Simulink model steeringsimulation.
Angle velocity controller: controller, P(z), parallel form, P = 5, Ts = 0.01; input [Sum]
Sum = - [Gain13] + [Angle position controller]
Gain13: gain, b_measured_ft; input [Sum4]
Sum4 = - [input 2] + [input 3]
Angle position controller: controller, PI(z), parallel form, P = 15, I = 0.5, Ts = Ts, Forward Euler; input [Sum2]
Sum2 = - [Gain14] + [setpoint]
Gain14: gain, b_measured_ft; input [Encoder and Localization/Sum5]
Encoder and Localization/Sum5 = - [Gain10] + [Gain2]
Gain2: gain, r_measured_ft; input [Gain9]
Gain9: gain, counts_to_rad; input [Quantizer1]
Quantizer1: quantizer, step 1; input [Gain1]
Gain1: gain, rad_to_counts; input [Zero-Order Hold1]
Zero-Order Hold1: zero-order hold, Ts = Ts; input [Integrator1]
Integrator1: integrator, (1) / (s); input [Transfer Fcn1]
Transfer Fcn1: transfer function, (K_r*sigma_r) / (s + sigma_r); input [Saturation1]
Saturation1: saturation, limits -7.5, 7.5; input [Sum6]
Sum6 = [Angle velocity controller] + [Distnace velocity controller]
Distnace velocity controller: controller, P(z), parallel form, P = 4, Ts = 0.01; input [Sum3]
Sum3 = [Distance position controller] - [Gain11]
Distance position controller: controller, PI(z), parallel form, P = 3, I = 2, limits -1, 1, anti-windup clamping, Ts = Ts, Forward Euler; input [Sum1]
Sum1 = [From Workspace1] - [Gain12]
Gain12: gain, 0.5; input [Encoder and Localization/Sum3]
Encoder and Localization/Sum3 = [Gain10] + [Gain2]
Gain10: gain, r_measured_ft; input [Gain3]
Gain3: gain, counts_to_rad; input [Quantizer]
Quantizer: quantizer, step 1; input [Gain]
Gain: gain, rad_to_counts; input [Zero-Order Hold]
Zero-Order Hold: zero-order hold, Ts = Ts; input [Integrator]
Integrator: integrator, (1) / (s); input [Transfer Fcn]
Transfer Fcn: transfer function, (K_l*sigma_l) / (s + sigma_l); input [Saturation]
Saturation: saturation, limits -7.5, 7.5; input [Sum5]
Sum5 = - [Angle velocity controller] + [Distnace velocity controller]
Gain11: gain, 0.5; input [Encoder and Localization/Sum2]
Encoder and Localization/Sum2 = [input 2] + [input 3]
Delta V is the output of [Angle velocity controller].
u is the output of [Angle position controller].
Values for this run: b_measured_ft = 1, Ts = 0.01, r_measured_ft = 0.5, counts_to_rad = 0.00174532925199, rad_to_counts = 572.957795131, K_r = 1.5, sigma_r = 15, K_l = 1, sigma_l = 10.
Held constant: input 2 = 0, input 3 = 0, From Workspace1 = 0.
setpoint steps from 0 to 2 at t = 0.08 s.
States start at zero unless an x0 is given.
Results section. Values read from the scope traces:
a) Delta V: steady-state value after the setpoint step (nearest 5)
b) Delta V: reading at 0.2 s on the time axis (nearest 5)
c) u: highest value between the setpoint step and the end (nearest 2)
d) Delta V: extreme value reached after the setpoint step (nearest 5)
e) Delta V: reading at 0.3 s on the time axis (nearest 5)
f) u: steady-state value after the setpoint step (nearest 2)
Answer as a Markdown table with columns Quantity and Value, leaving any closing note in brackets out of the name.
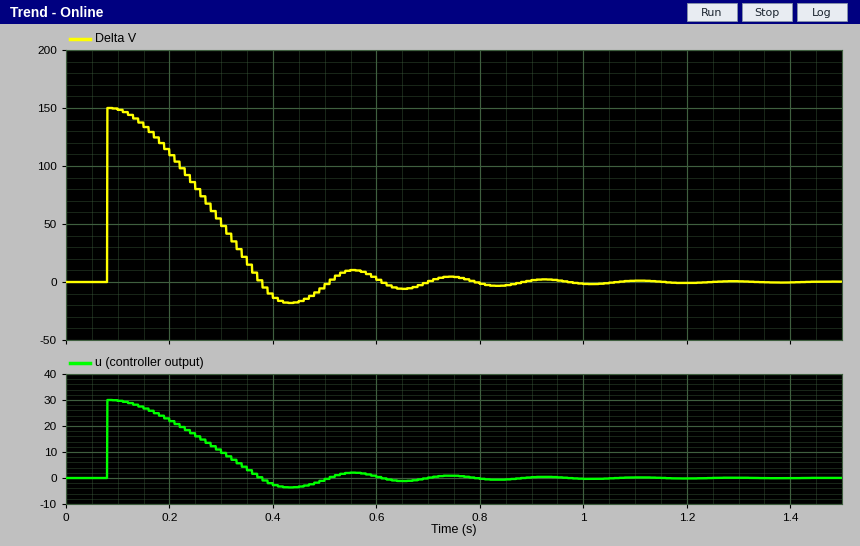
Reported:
| Quantity | Value |
|---|---|
| Delta V: steady-state value after the setpoint step | 0 |
| Delta V: reading at 0.2 s on the time axis | 110 |
| u: highest value between the setpoint step and the end | 30 |
| Delta V: extreme value reached after the setpoint step | 150 |
| Delta V: reading at 0.3 s on the time axis | 50 |
| u: steady-state value after the setpoint step | 0 |
